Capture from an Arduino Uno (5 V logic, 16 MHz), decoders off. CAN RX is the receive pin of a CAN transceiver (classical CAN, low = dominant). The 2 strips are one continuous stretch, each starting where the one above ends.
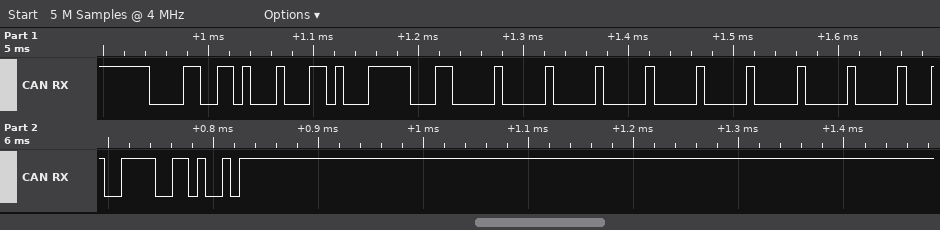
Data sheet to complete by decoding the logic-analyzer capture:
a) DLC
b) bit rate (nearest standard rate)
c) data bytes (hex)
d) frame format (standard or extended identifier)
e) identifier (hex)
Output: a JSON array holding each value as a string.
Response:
["8", "125 kbit/s", "D1 F3 00 00 00 00 00 00", "standard", "0x0CD"]
